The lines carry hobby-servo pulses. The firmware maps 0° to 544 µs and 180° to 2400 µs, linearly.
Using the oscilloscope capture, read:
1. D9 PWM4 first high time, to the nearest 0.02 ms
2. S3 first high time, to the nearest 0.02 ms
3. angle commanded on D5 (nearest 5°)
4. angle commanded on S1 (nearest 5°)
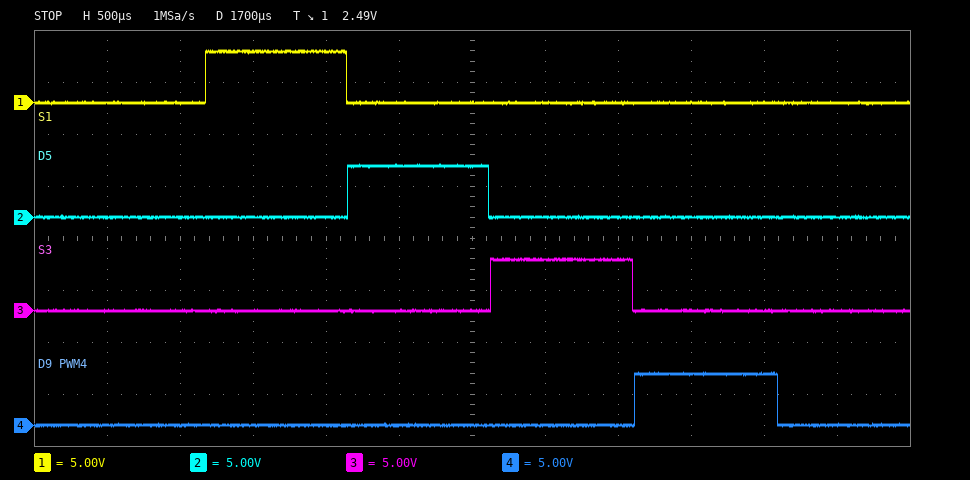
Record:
0.98 ms
0.98 ms
40°
40°
